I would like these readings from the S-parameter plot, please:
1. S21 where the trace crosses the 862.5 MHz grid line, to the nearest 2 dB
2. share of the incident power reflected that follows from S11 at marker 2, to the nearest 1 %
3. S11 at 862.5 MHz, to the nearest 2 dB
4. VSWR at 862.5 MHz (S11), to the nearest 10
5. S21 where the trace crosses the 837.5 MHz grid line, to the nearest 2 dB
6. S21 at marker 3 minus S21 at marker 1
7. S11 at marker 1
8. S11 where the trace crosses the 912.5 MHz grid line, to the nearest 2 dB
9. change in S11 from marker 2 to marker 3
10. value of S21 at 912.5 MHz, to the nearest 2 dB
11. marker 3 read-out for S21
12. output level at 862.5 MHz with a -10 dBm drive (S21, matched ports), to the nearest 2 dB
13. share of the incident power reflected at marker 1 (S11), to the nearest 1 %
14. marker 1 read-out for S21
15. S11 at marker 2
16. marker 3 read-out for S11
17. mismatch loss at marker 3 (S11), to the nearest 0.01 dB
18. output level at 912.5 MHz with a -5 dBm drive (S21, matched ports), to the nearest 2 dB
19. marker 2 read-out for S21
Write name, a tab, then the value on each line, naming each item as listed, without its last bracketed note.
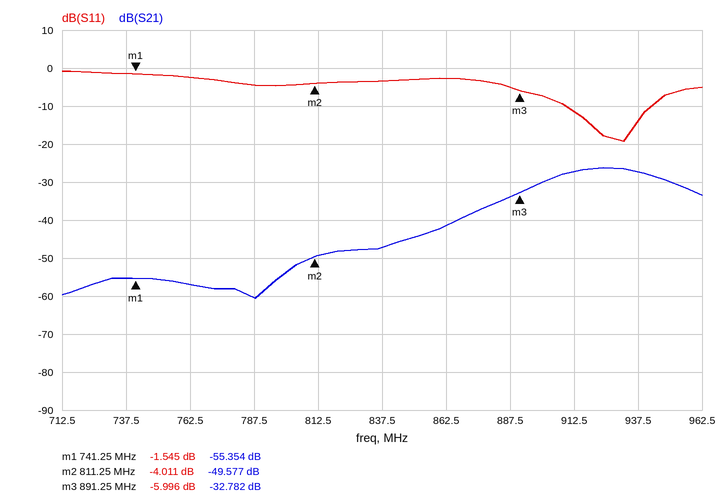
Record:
S21 where the trace crosses the 862.5 MHz grid line, to the nearest 2 dB	-42 dB
share of the incident power reflected that follows from S11 at marker 2, to the nearest 1 %	40 %
S11 at 862.5 MHz, to the nearest 2 dB	-2 dB
VSWR at 862.5 MHz (S11), to the nearest 10	10
S21 where the trace crosses the 837.5 MHz grid line, to the nearest 2 dB	-48 dB
S21 at marker 3 minus S21 at marker 1	22.572 dB
S11 at marker 1	-1.545 dB
S11 where the trace crosses the 912.5 MHz grid line, to the nearest 2 dB	-12 dB
change in S11 from marker 2 to marker 3	-1.985 dB
value of S21 at 912.5 MHz, to the nearest 2 dB	-28 dB
marker 3 read-out for S21	-32.782 dB
output level at 862.5 MHz with a -10 dBm drive (S21, matched ports), to the nearest 2 dB	-52 dBm
share of the incident power reflected at marker 1 (S11), to the nearest 1 %	70 %
marker 1 read-out for S21	-55.354 dB
S11 at marker 2	-4.011 dB
marker 3 read-out for S11	-5.996 dB
mismatch loss at marker 3 (S11), to the nearest 0.01 dB	1.26 dB
output level at 912.5 MHz with a -5 dBm drive (S21, matched ports), to the nearest 2 dB	-32 dBm
marker 2 read-out for S21	-49.577 dB
